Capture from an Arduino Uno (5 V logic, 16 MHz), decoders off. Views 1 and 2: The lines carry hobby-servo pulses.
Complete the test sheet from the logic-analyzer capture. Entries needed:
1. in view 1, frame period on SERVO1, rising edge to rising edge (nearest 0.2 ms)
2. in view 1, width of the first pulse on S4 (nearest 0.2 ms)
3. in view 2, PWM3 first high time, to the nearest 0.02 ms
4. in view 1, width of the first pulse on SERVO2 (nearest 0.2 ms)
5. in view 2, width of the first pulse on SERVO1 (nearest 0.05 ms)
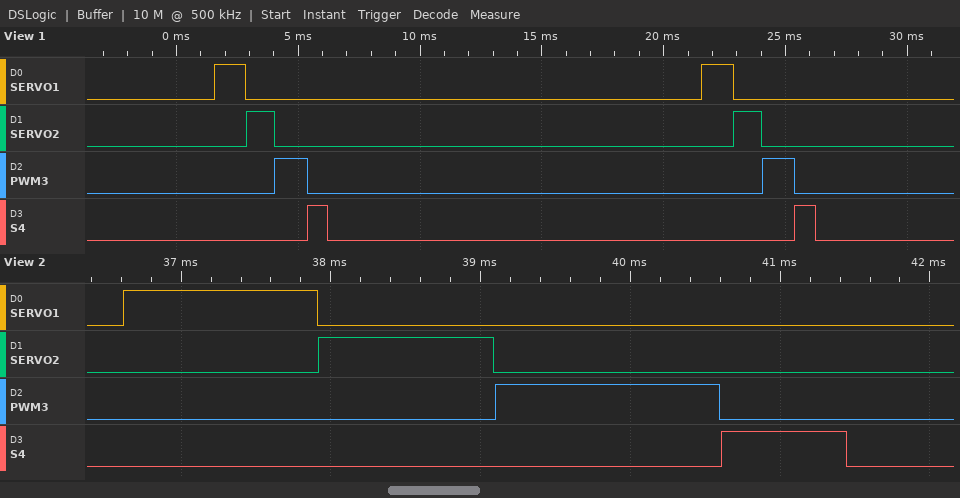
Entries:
20.0 ms
0.8 ms
1.50 ms
1.2 ms
1.30 ms
